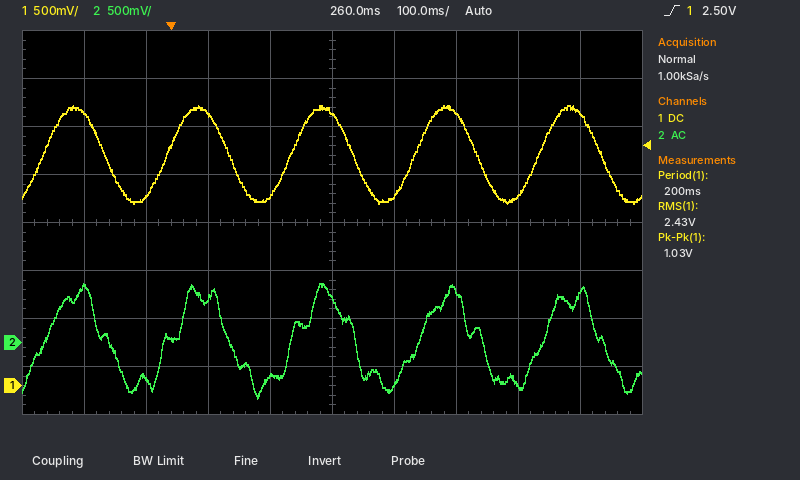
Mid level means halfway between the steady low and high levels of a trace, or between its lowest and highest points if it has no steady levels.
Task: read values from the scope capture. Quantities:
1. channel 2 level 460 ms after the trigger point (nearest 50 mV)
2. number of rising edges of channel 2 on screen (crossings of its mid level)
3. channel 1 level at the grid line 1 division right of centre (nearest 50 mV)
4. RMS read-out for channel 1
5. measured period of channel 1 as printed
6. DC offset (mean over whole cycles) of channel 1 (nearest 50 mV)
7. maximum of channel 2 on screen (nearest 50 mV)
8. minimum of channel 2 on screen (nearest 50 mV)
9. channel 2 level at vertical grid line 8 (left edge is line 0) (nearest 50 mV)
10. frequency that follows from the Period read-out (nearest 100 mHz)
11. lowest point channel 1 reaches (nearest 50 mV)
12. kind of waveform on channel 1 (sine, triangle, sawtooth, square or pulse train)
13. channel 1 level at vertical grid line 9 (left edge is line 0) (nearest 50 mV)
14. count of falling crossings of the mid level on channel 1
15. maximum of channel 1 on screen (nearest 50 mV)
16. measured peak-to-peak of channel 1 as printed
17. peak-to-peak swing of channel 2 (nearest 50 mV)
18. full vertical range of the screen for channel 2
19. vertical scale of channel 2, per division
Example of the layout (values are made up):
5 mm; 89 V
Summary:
550 mV; 5; 2.00 V; 2.43 V; 200 ms; 2.40 V; 600 mV; -600 mV; -450 mV; 5.0 Hz; 1.90 V; sine; 2.85 V; 5; 2.90 V; 1.03 V; 1.20 V; 4 V; 500 mV
